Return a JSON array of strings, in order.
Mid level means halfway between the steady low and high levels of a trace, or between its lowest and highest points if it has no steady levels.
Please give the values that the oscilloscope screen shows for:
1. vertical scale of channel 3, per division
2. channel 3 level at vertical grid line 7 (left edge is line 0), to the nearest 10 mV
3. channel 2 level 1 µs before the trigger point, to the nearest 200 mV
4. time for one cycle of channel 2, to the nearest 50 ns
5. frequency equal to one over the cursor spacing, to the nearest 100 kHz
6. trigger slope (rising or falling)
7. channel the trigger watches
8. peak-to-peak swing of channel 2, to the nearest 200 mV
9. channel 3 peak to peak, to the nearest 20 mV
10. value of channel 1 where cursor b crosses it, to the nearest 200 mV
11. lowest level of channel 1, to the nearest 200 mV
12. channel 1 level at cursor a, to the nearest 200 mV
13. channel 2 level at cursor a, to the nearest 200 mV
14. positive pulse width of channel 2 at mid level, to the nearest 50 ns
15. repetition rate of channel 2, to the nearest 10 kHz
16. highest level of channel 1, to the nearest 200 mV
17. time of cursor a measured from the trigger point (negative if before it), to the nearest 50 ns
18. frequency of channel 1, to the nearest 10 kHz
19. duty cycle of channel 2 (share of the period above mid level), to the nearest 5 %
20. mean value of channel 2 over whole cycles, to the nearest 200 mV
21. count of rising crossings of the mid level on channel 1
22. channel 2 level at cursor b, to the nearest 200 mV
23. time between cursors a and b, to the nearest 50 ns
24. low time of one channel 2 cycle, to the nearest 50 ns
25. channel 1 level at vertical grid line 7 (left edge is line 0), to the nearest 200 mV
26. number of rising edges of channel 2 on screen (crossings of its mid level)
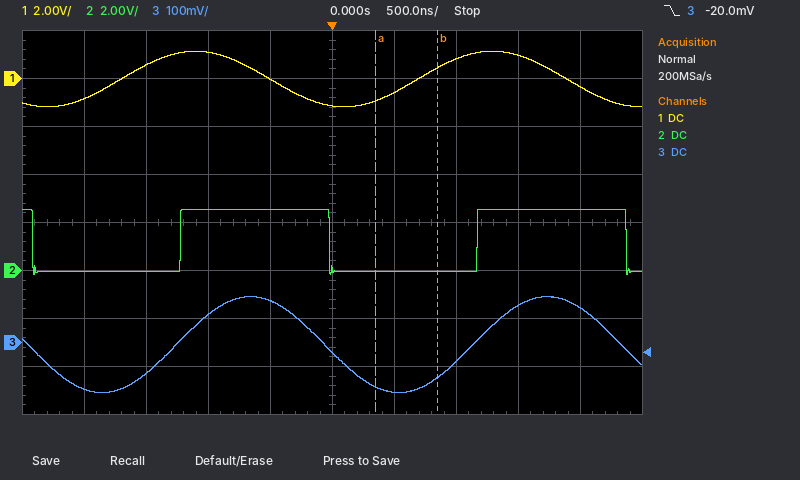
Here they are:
["100 mV", "-40 mV", "2.6 V", "2.40 µs", "2.0 MHz", "falling", "channel 3", "2.8 V", "200 mV", "400 mV", "-1.2 V", "-1.0 V", "0.0 V", "1.20 µs", "420 kHz", "1.2 V", "+350 ns", "420 kHz", "50 %", "1.2 V", "2", "0.0 V", "500 ns", "1.20 µs", "800 mV", "2"]
